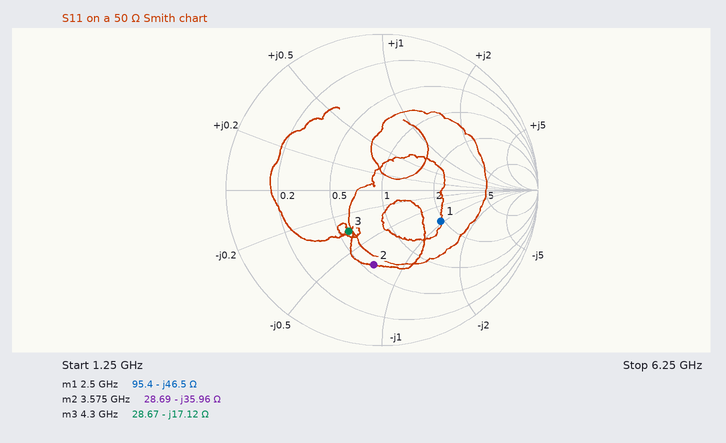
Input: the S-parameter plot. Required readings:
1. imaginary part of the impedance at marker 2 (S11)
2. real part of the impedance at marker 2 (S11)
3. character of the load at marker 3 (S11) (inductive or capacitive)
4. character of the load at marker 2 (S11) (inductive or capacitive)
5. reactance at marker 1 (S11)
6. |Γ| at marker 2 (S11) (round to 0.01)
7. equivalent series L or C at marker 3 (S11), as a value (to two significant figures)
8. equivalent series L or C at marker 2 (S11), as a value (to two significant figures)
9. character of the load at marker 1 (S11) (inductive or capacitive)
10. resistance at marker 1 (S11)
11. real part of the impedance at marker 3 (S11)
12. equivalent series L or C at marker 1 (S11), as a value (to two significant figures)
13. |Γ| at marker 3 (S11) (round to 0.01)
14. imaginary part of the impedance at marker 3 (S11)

-35.96 Ω
28.69 Ω
capacitive
capacitive
-46.5 Ω
0.48
2.2 pF
1.2 pF
capacitive
95.4 Ω
28.67 Ω
1.4 pF
0.34
-17.12 Ω
